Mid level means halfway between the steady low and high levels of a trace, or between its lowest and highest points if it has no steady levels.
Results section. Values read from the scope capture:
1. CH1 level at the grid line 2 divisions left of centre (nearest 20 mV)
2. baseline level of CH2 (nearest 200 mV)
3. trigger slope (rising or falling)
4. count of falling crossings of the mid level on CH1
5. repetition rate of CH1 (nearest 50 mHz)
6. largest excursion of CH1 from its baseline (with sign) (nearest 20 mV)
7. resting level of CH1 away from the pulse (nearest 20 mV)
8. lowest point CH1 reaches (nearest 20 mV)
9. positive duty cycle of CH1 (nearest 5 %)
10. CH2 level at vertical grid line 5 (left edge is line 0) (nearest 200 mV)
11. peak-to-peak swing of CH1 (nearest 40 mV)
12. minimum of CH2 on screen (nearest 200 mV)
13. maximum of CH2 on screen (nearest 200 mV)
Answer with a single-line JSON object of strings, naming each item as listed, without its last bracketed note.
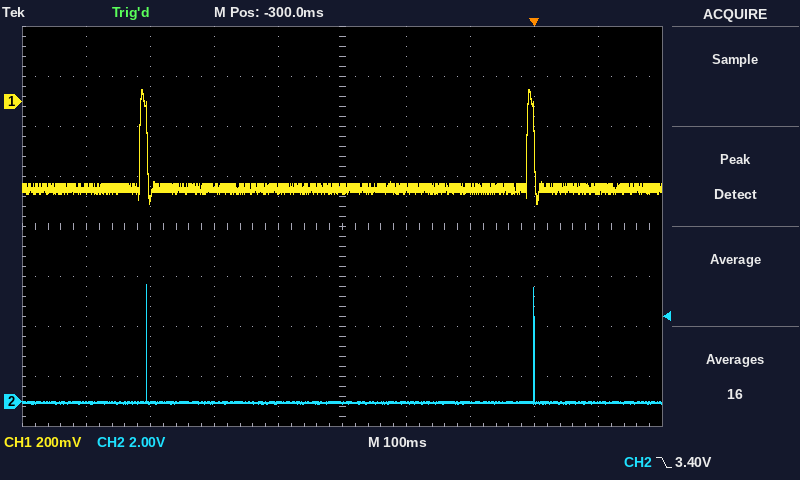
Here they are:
{"CH1 level at the grid line 2 divisions left of centre": "-340 mV", "baseline level of CH2": "0.0 V", "trigger slope": "falling", "count of falling crossings of the mid level on CH1": "2", "repetition rate of CH1": "1.65 Hz", "largest excursion of CH1 from its baseline (with sign)": "+400 mV", "resting level of CH1 away from the pulse": "-340 mV", "lowest point CH1 reaches": "-400 mV", "positive duty cycle of CH1": "0 %", "CH2 level at vertical grid line 5 (left edge is line 0)": "0.0 V", "peak-to-peak swing of CH1": "440 mV", "minimum of CH2 on screen": "0.0 V", "maximum of CH2 on screen": "4.6 V"}
